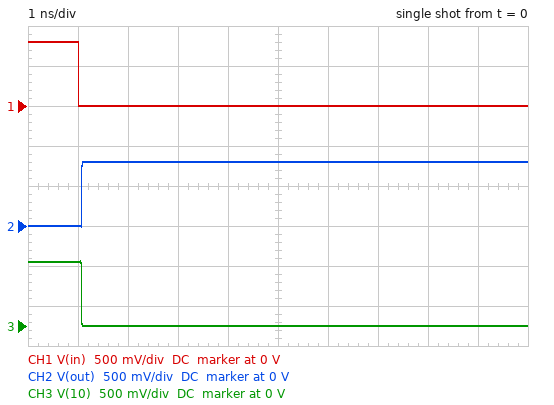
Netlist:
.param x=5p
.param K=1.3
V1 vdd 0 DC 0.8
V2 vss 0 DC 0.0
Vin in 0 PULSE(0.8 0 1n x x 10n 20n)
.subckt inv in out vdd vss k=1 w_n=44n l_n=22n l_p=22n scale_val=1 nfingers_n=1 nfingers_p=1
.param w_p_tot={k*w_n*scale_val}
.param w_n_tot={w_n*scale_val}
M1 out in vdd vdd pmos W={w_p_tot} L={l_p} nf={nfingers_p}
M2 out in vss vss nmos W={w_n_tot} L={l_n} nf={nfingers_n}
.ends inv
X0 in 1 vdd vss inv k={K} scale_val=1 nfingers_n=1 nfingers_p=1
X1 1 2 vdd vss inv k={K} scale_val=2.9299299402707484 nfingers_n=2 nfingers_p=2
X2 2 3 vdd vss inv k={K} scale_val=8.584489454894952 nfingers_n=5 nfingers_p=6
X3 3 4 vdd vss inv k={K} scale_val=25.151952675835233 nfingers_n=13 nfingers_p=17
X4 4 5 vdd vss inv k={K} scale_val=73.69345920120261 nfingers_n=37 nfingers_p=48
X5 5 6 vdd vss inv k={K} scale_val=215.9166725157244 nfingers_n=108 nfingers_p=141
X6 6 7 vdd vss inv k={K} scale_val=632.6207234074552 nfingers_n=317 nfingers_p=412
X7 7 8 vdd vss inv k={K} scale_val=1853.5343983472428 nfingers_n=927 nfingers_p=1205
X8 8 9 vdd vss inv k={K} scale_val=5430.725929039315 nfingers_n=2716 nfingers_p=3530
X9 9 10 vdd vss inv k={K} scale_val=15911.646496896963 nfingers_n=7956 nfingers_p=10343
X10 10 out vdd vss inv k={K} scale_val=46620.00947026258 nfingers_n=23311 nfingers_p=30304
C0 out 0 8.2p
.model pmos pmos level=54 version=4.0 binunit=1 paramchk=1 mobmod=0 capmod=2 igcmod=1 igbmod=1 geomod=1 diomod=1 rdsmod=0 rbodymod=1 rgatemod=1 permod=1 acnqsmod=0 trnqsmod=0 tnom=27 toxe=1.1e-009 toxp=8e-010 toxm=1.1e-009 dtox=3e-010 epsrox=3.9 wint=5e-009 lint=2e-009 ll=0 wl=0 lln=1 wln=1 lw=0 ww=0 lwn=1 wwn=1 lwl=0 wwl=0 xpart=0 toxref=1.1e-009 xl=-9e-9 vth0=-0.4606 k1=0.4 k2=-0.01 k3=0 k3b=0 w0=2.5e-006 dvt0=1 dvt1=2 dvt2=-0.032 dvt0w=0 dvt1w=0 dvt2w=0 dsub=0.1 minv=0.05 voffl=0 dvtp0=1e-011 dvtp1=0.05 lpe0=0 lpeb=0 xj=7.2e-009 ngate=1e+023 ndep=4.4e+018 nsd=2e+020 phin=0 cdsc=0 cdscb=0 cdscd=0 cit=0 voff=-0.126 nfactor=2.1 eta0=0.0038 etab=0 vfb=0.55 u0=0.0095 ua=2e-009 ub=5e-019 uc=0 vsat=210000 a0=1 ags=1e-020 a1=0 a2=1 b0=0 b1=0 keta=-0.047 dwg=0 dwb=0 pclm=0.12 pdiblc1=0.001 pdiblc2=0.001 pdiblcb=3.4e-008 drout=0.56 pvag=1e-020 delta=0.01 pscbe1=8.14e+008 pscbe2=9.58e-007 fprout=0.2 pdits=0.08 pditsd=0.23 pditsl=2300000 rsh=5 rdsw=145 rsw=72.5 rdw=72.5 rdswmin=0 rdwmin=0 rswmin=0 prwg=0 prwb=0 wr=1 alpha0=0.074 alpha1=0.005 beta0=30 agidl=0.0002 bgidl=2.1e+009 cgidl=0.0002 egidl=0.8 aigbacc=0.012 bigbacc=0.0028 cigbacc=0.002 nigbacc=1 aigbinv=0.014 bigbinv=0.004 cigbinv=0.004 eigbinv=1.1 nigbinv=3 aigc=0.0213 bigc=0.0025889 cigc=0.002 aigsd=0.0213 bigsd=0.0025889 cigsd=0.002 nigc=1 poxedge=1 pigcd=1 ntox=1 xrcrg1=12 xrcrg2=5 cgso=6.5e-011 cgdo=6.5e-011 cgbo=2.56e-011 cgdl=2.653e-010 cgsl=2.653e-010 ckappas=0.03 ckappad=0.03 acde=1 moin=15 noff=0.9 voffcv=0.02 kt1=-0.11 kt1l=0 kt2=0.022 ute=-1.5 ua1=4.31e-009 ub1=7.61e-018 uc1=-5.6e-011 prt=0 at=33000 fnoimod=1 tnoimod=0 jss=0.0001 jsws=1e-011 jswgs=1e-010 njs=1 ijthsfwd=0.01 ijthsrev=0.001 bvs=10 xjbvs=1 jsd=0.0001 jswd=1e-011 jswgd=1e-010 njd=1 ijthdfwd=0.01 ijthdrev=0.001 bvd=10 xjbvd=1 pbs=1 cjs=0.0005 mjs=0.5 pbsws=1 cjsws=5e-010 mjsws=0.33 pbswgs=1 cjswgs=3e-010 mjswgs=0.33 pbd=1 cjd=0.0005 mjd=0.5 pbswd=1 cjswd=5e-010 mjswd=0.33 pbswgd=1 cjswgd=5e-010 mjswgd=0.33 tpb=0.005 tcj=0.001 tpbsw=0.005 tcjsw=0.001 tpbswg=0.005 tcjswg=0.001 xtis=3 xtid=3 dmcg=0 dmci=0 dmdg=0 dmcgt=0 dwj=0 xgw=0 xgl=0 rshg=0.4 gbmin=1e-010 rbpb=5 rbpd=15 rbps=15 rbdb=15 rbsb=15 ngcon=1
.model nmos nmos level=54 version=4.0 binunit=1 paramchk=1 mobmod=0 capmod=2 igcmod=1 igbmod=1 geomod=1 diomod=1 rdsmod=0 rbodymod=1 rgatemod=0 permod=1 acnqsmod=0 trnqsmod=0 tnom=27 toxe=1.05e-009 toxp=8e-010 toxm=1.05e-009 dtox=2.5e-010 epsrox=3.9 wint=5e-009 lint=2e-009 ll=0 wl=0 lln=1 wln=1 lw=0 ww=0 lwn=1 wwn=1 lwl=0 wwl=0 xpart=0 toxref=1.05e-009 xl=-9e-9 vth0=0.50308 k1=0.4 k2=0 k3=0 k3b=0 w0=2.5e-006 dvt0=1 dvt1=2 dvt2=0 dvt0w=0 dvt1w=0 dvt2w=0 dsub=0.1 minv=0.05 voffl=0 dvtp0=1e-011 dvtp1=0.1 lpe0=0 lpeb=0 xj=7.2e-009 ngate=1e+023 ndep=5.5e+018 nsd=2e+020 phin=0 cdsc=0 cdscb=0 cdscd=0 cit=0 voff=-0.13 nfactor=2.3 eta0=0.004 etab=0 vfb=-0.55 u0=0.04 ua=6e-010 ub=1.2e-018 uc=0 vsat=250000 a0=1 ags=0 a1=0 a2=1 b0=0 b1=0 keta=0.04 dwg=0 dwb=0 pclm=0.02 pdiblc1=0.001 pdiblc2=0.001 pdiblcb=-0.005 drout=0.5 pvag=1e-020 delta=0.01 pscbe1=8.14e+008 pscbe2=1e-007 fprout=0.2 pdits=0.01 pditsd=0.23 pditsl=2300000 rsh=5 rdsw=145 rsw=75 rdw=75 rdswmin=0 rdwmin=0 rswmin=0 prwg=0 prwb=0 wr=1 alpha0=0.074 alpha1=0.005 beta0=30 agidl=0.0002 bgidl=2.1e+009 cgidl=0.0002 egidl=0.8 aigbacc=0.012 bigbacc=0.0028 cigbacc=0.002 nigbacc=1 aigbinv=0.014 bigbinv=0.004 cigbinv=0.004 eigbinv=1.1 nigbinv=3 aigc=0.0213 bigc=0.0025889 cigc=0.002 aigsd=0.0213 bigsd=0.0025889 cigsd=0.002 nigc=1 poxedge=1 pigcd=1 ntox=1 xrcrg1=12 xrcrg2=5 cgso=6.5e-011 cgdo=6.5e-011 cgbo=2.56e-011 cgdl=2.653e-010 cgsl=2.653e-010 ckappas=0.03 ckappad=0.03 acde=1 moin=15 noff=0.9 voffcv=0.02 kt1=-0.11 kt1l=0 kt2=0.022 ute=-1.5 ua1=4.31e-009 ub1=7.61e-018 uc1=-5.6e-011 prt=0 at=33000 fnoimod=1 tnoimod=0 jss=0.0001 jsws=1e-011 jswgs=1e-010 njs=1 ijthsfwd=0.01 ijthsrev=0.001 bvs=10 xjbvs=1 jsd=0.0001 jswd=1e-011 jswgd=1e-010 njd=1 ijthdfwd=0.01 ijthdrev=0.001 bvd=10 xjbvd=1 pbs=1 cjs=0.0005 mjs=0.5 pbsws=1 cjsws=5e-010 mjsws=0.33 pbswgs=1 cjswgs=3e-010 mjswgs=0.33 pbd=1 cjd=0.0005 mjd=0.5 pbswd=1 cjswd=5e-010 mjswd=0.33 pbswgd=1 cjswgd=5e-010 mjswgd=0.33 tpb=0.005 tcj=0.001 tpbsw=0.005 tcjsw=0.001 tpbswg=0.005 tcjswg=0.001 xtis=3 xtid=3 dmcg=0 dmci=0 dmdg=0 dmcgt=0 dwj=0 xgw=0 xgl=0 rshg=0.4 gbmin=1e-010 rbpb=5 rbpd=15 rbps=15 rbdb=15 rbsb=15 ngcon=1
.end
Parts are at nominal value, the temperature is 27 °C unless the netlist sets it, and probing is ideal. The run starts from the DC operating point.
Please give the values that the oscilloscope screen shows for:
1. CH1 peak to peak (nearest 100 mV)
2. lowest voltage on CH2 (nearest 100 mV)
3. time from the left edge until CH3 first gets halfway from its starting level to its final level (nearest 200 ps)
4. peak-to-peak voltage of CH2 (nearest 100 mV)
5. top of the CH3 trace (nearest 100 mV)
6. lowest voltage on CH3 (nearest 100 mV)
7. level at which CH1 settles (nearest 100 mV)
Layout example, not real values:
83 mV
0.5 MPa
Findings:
800 mV
0 V
1.0 ns
800 mV
800 mV
0 V
0 V
